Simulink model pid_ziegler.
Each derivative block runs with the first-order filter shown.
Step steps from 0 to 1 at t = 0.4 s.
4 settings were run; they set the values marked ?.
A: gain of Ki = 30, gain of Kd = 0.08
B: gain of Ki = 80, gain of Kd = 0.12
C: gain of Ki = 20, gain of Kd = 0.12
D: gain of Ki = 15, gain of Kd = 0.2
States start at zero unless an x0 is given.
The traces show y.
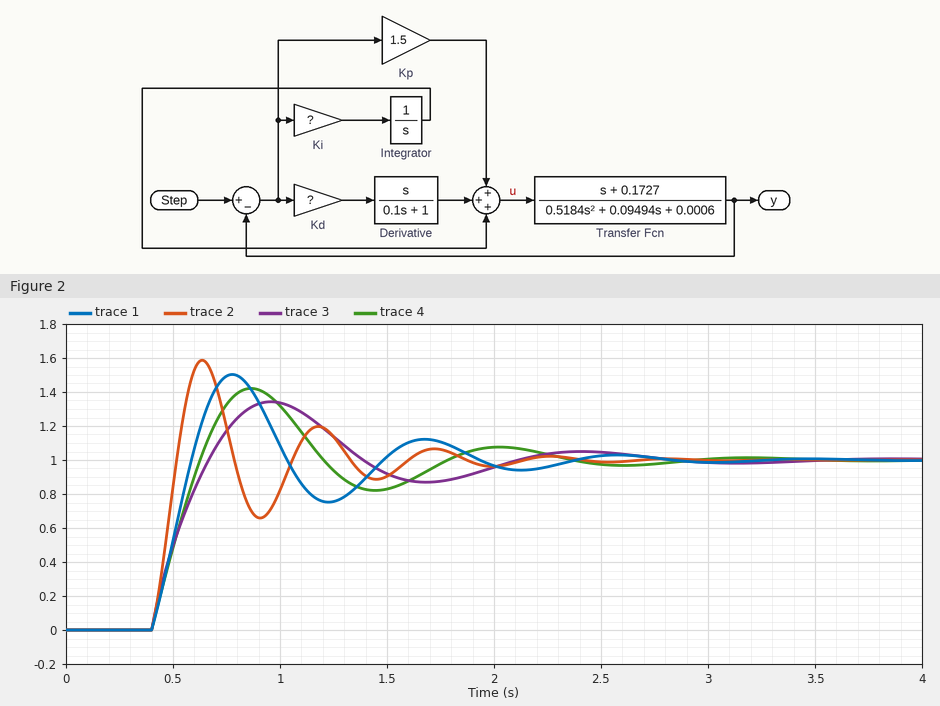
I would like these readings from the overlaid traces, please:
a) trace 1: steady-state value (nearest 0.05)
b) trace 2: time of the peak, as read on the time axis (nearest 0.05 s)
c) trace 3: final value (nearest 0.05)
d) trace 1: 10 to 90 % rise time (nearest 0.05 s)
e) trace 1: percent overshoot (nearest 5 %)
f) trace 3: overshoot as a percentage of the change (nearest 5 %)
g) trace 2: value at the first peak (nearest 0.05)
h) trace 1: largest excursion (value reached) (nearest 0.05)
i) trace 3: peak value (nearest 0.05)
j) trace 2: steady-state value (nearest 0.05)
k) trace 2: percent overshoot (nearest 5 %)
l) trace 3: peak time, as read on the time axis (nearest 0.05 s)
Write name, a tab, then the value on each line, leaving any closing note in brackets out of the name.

trace 1: steady-state value	1.00
trace 2: time of the peak, as read on the time axis	0.65 s
trace 3: final value	1.00
trace 1: 10 to 90 % rise time	0.15 s
trace 1: percent overshoot	50 %
trace 3: overshoot as a percentage of the change	35 %
trace 2: value at the first peak	1.60
trace 1: largest excursion (value reached)	1.50
trace 3: peak value	1.35
trace 2: steady-state value	1.00
trace 2: percent overshoot	60 %
trace 3: peak time, as read on the time axis	0.95 s
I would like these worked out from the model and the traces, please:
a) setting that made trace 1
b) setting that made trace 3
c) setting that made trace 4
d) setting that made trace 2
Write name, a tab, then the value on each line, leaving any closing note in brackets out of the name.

setting that made trace 1	A
setting that made trace 3	D
setting that made trace 4	C
setting that made trace 2	B
